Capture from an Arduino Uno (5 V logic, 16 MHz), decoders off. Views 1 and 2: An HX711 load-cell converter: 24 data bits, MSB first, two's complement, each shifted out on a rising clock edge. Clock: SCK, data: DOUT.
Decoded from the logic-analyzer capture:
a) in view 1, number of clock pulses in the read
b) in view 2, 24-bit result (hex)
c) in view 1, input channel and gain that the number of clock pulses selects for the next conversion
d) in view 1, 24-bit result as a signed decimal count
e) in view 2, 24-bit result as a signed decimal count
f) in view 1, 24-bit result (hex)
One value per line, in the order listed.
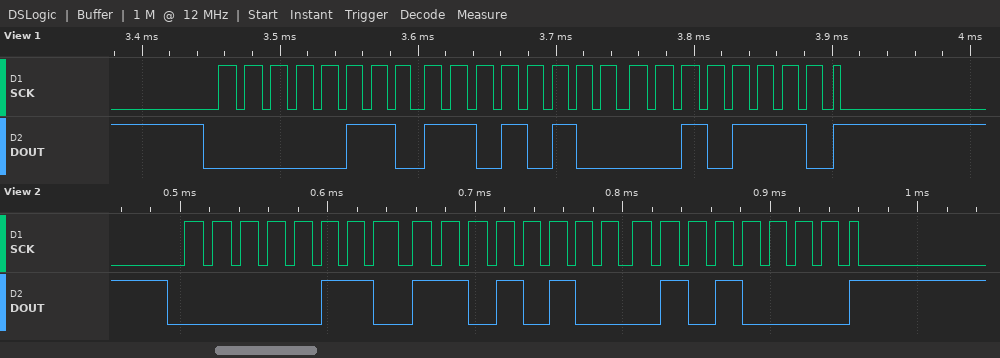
25
0x06D450
channel A, gain 128
447534
447568
0x06D42E
